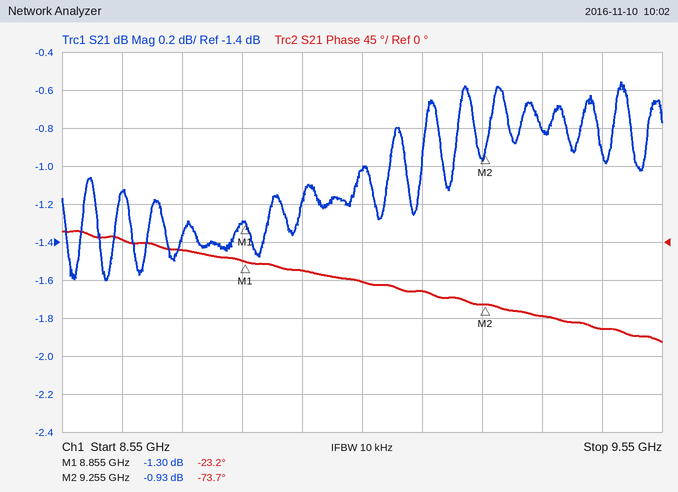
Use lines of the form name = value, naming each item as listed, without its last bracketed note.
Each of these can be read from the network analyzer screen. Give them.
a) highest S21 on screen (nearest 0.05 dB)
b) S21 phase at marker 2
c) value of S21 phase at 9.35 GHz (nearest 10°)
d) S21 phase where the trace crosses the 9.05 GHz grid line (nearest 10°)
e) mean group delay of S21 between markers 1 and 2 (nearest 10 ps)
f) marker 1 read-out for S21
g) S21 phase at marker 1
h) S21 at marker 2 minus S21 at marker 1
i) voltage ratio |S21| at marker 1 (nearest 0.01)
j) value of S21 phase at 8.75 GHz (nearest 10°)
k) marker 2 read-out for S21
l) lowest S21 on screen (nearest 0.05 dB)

highest S21 on screen = -0.55 dB
S21 phase at marker 2 = -73.7°
value of S21 phase at 9.35 GHz = -90°
S21 phase where the trace crosses the 9.05 GHz grid line = -50°
mean group delay of S21 between markers 1 and 2 = 350 ps
marker 1 read-out for S21 = -1.30 dB
S21 phase at marker 1 = -23.2°
S21 at marker 2 minus S21 at marker 1 = 0.37 dB
voltage ratio |S21| at marker 1 = 0.86
value of S21 phase at 8.75 GHz = -10°
marker 2 read-out for S21 = -0.93 dB
lowest S21 on screen = -1.60 dB
